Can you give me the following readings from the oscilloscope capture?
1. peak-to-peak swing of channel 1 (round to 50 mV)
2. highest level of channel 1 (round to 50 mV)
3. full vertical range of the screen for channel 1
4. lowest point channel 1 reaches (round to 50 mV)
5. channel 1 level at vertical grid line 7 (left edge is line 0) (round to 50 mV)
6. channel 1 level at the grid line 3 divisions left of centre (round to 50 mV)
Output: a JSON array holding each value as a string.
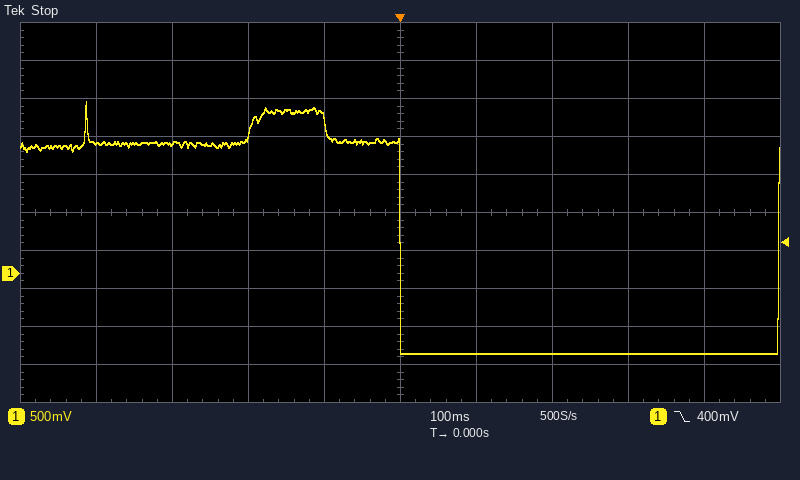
["3.30 V", "2.25 V", "5 V", "-1.05 V", "-1.05 V", "1.70 V"]
